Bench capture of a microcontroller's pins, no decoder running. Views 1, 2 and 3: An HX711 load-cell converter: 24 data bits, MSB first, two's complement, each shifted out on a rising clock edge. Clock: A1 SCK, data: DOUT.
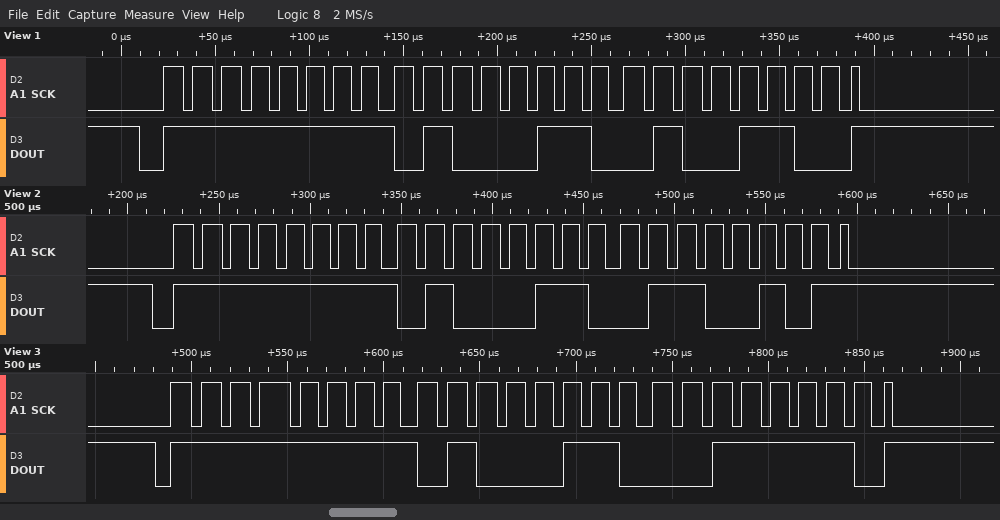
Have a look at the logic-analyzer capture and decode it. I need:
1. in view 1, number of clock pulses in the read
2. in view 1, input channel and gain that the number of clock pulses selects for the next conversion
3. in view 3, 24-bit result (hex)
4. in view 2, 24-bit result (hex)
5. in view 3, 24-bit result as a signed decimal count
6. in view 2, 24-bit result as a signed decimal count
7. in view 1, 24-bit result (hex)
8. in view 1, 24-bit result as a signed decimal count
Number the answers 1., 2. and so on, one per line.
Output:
1. 25
2. channel A, gain 128
3. 0xFF463E
4. 0xFF4665
5. -47554
6. -47515
7. 0xFF464C
8. -47540
